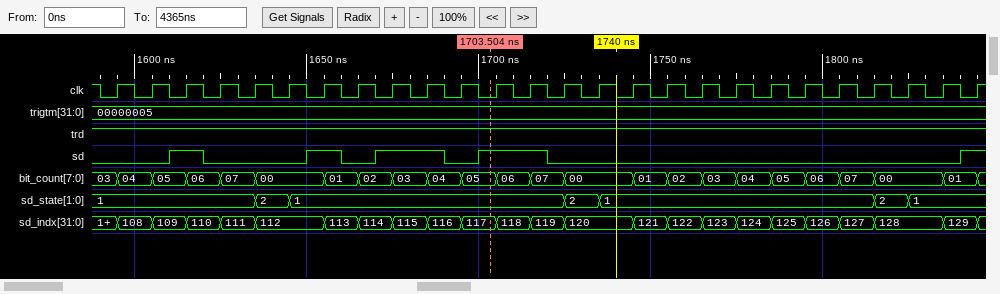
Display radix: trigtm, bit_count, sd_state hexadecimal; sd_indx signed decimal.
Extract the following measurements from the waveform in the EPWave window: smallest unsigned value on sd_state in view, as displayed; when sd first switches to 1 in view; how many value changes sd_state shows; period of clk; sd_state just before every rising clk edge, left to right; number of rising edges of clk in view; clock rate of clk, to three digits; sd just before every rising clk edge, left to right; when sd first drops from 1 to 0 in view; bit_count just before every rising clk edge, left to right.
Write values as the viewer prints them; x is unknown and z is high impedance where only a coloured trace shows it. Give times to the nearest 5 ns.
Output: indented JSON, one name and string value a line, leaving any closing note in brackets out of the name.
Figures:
{
  "smallest unsigned value on sd_state in view, as displayed": "1",
  "when sd first switches to 1 in view": "1610 ns",
  "how many value changes sd_state shows": "6",
  "period of clk": "10 ns",
  "sd_state just before every rising clk edge, left to right": "1, 1, 1, 1, 1, 2, 1, 1, 1, 1, 1, 1, 1, 1, 2, 1, 1, 1, 1, 1, 1, 1, 1, 2, 1, 1",
  "number of rising edges of clk in view": "26",
  "clock rate of clk, to three digits": "100 MHz",
  "sd just before every rising clk edge, left to right": "0 0 1 0 0 0 1 0 1 1 0 1 1 0 0 0 0 0 0 0 0 0 0 0 0 1",
  "when sd first drops from 1 to 0 in view": "1620 ns",
  "bit_count just before every rising clk edge, left to right": "03, 04, 05, 06, 07, 00, 00, 01, 02, 03, 04, 05, 06, 07, 00, 00, 01, 02, 03, 04, 05, 06, 07, 00, 00, 01"
}
